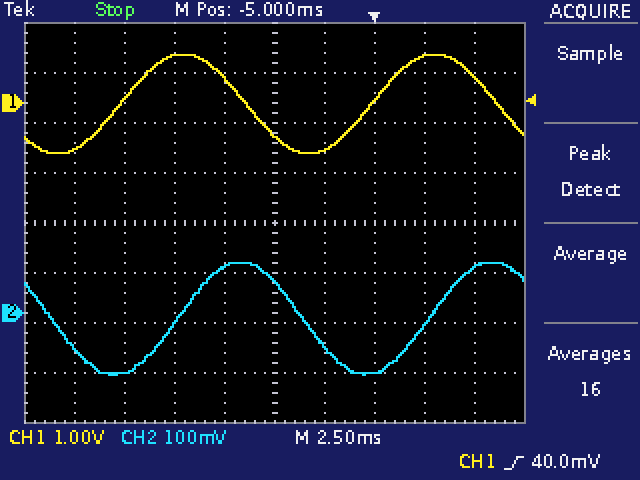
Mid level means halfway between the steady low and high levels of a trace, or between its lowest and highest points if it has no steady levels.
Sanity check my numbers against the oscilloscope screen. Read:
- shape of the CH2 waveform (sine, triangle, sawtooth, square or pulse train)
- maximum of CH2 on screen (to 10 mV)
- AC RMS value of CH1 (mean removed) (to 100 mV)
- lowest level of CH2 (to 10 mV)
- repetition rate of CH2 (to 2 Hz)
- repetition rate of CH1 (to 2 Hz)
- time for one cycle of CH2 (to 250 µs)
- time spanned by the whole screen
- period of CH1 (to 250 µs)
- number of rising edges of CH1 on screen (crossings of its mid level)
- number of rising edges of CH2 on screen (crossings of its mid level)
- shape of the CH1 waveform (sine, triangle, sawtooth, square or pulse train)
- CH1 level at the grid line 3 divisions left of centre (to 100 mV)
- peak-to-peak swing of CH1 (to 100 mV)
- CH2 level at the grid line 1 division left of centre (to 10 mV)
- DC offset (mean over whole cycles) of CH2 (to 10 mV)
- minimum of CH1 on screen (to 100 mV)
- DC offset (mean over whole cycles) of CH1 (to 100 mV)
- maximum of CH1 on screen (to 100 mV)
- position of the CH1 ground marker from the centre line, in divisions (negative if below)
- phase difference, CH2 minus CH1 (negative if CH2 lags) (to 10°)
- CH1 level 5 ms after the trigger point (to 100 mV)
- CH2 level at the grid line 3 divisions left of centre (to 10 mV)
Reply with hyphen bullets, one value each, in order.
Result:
- sine
- 100 mV
- 700 mV
- -120 mV
- 80 Hz
- 80 Hz
- 12.50 ms
- 25 ms
- 12.50 ms
- 2
- 2
- sine
- 100 mV
- 2.0 V
- 90 mV
- -10 mV
- -1.0 V
- 0.0 V
- 1.0 V
- +2.4 div
- -80°
- 500 mV
- -120 mV
